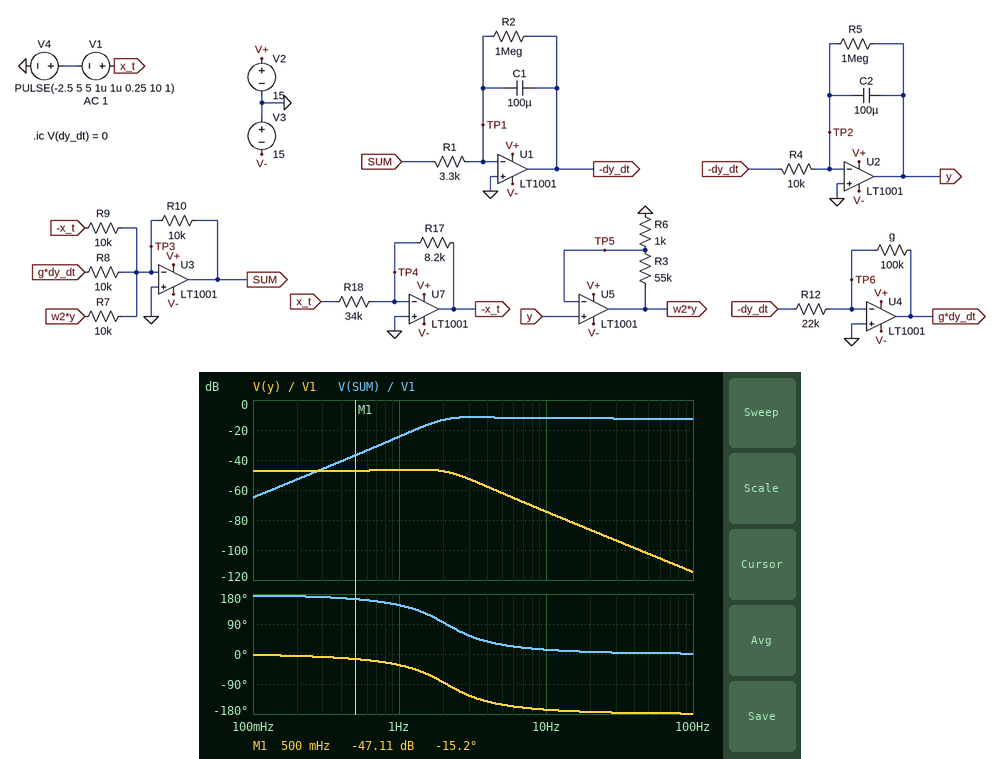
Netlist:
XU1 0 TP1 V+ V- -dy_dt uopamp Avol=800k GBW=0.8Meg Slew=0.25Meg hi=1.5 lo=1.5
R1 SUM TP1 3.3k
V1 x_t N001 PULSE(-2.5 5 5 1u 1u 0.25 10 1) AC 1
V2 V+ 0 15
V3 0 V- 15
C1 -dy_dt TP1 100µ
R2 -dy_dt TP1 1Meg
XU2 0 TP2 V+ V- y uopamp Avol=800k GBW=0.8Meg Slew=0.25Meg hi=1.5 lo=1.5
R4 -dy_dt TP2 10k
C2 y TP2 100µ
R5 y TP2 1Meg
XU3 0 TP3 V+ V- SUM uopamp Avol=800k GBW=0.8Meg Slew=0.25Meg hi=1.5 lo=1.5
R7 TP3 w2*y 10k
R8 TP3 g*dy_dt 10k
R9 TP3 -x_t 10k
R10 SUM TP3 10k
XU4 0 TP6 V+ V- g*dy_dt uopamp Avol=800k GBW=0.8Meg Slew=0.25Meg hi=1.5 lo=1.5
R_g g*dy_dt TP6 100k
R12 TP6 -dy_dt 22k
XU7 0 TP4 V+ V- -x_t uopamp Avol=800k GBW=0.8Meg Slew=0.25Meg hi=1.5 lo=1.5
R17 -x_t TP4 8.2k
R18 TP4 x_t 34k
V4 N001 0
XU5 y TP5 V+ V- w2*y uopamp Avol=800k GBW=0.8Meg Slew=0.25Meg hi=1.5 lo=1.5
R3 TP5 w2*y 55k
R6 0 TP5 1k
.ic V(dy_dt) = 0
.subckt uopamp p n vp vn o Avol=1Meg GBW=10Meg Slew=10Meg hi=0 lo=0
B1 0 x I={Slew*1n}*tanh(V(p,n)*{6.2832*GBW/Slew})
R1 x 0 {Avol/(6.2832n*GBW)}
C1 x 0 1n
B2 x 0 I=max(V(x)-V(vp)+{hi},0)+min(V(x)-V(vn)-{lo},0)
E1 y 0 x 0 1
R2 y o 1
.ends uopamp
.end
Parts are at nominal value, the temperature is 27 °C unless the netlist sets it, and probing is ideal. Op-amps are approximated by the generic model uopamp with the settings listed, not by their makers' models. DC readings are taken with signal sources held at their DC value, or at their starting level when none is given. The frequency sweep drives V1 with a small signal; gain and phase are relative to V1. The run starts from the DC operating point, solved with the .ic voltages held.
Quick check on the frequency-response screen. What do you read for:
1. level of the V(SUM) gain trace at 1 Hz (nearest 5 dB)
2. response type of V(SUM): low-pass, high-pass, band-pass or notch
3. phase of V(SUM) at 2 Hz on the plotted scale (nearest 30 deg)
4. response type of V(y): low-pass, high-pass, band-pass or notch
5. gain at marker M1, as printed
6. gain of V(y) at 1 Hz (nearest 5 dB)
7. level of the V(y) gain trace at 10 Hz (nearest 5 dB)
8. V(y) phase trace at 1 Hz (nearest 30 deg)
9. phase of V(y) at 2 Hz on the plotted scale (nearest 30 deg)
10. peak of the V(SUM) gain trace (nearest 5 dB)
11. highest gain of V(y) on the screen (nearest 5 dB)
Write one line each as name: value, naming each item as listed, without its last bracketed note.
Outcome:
level of the V(SUM) gain trace at 1 Hz: -25 dB
response type of V(SUM): low-pass, high-pass, band-pass or notch: high-pass
phase of V(SUM) at 2 Hz on the plotted scale: 90 deg
response type of V(y): low-pass, high-pass, band-pass or notch: low-pass
gain at marker M1, as printed: -47.11 dB
gain of V(y) at 1 Hz: -45 dB
level of the V(y) gain trace at 10 Hz: -75 dB
V(y) phase trace at 1 Hz: -30 deg
phase of V(y) at 2 Hz on the plotted scale: -90 deg
peak of the V(SUM) gain trace: -10 dB
highest gain of V(y) on the screen: -45 dB
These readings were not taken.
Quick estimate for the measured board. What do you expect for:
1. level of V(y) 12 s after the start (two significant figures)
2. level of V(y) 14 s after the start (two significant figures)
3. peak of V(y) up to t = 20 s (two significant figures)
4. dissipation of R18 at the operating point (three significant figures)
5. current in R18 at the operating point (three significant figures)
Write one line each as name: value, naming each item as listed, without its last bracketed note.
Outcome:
level of V(y) 12 s after the start: -11 mV
level of V(y) 14 s after the start: -11 mV
peak of V(y) up to t = 20 s: 26 mV
dissipation of R18 at the operating point: 184 µW
current in R18 at the operating point: 73.5 µA
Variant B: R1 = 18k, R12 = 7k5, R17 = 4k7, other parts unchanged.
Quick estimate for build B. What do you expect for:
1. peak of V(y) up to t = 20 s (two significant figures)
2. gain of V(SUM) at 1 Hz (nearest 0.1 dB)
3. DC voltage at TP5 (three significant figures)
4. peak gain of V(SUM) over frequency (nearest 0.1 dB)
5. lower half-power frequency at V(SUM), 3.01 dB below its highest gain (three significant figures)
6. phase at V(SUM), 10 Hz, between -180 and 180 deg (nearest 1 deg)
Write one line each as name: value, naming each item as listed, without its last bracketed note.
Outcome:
peak of V(y) up to t = 20 s: 5.1 mV
gain of V(SUM) at 1 Hz: -18.8 dB
DC voltage at TP5: -6.16 mV
peak gain of V(SUM) over frequency: -17.1 dB
lower half-power frequency at V(SUM), 3.01 dB below its highest gain: 844 mHz
phase at V(SUM), 10 Hz, between -180 and 180 deg: 7 deg
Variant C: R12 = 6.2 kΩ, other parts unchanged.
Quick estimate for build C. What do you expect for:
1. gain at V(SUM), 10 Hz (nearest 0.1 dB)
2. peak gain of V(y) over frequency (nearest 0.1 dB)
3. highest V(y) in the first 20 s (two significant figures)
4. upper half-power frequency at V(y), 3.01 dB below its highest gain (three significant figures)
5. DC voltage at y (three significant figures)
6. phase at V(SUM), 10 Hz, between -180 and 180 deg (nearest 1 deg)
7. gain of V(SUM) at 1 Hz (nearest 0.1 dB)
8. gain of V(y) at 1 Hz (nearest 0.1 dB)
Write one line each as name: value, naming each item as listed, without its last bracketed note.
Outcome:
gain at V(SUM), 10 Hz: -14.2 dB
peak gain of V(y) over frequency: -47.3 dB
highest V(y) in the first 20 s: 8.1 mV
upper half-power frequency at V(y), 3.01 dB below its highest gain: 596 mHz
DC voltage at y: -10.7 mV
phase at V(SUM), 10 Hz, between -180 and 180 deg: 39 deg
gain of V(SUM) at 1 Hz: -30.9 dB
gain of V(y) at 1 Hz: -53.2 dB
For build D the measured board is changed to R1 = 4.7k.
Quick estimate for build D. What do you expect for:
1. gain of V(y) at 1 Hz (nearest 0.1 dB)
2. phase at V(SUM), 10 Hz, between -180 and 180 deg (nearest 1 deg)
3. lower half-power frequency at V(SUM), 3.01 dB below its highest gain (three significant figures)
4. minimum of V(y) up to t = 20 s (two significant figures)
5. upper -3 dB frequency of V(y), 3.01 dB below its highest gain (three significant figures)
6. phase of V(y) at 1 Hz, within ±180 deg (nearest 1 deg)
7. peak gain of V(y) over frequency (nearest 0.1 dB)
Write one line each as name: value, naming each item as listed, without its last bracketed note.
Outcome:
gain of V(y) at 1 Hz: -45.8 dB
phase at V(SUM), 10 Hz, between -180 and 180 deg: 9 deg
lower half-power frequency at V(SUM), 3.01 dB below its highest gain: 1.47 Hz
minimum of V(y) up to t = 20 s: -19 mV
upper -3 dB frequency of V(y), 3.01 dB below its highest gain: 2.06 Hz
phase of V(y) at 1 Hz, within ±180 deg: -37 deg
peak gain of V(y) over frequency: -45.3 dB
